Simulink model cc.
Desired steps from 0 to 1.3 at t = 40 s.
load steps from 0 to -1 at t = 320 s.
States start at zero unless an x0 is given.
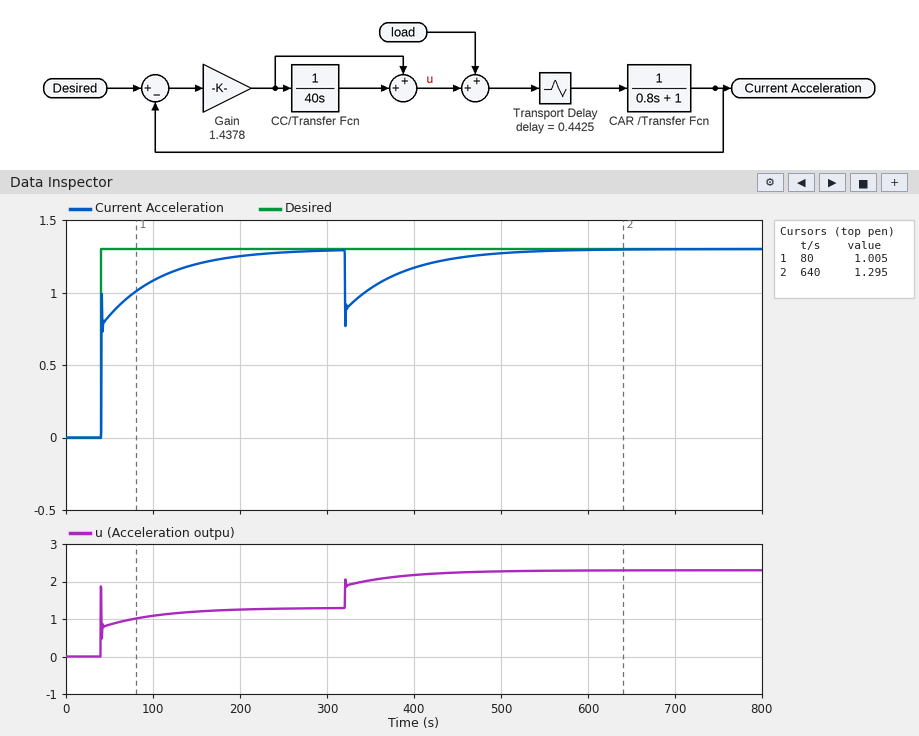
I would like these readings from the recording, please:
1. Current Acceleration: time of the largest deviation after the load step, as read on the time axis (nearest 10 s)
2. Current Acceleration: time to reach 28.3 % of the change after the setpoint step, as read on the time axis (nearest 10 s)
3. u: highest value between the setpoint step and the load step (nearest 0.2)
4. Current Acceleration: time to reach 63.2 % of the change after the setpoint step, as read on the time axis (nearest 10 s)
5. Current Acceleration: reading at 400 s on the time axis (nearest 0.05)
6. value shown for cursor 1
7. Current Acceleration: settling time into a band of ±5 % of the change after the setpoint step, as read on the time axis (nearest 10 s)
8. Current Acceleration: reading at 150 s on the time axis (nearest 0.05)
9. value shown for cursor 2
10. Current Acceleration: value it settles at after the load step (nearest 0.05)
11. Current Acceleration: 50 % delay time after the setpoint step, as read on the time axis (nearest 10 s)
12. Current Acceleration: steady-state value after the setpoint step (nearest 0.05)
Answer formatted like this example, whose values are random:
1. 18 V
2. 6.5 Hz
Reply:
1. 320 s
2. 40 s
3. 1.8
4. 40 s
5. 1.15
6. 1.005
7. 180 s
8. 1.20
9. 1.295
10. 1.30
11. 40 s
12. 1.30
